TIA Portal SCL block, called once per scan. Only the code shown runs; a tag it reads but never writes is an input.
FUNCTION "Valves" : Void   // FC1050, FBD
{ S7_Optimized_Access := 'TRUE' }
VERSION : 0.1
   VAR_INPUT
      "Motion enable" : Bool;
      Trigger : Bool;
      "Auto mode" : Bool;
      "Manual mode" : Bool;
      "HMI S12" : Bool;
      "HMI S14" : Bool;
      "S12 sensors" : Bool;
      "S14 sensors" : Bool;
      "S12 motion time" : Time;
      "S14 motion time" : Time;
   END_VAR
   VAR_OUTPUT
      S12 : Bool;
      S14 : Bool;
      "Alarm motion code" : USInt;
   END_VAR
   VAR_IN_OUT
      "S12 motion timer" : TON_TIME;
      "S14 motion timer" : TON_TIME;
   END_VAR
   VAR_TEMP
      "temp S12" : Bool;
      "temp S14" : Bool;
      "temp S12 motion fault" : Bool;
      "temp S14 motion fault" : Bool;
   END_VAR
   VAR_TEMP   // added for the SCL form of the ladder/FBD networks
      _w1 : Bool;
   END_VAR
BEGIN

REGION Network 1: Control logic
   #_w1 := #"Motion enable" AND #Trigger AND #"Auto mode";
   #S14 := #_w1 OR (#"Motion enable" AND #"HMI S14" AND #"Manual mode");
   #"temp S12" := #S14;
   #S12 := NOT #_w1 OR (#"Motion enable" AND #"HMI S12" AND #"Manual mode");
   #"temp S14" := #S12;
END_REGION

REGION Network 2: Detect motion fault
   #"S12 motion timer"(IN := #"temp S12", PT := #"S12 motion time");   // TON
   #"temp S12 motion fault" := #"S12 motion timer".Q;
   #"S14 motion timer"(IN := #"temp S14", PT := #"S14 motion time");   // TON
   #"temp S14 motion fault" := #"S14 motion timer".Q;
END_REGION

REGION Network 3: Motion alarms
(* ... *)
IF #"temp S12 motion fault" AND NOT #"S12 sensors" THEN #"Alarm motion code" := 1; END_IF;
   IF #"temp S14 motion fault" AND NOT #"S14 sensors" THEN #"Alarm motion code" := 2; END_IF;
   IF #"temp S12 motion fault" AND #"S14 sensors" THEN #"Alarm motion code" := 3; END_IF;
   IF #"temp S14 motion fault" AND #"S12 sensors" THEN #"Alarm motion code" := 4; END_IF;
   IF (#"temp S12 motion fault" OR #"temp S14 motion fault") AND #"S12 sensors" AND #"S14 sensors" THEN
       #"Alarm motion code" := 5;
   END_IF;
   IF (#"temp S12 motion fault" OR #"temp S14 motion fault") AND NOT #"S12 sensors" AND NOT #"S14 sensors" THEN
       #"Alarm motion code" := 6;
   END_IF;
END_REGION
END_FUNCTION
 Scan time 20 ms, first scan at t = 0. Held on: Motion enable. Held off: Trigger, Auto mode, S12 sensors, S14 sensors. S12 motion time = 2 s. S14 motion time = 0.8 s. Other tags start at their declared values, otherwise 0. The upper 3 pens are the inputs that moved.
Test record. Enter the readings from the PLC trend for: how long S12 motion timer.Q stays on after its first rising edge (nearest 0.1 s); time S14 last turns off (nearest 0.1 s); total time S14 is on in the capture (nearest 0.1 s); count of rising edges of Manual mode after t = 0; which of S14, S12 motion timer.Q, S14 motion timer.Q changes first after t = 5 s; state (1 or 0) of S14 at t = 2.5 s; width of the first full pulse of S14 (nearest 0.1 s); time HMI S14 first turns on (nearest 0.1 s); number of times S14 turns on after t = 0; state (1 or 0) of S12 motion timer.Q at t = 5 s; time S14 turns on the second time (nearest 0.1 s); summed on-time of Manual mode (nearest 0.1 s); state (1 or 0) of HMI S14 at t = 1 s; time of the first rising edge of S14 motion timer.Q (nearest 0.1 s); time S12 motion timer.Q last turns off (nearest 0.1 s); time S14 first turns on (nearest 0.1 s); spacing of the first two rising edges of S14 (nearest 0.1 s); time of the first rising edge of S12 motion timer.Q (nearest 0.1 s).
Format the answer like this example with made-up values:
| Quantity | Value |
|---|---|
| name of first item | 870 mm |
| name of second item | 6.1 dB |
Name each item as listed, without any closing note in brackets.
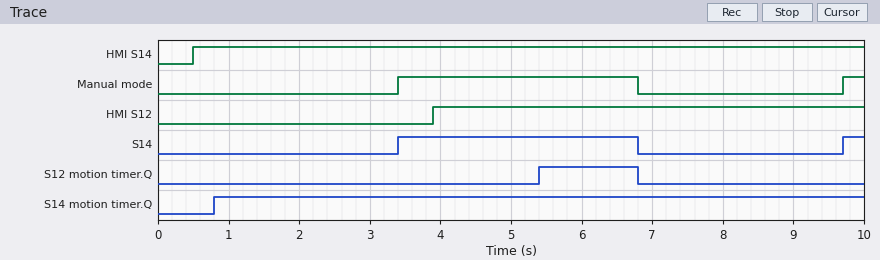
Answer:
| Quantity | Value |
|---|---|
| how long S12 motion timer.Q stays on after its first rising edge | 1.4 s |
| time S14 last turns off | 6.8 s |
| total time S14 is on in the capture | 3.7 s |
| count of rising edges of Manual mode after t = 0 | 2 |
| which of S14, S12 motion timer.Q, S14 motion timer.Q changes first after t = 5 s | S12 motion timer.Q |
| state (1 or 0) of S14 at t = 2.5 s | 0 |
| width of the first full pulse of S14 | 3.4 s |
| time HMI S14 first turns on | 0.5 s |
| number of times S14 turns on after t = 0 | 2 |
| state (1 or 0) of S12 motion timer.Q at t = 5 s | 0 |
| time S14 turns on the second time | 9.7 s |
| summed on-time of Manual mode | 3.7 s |
| state (1 or 0) of HMI S14 at t = 1 s | 1 |
| time of the first rising edge of S14 motion timer.Q | 0.8 s |
| time S12 motion timer.Q last turns off | 6.8 s |
| time S14 first turns on | 3.4 s |
| spacing of the first two rising edges of S14 | 6.3 s |
| time of the first rising edge of S12 motion timer.Q | 5.4 s |
